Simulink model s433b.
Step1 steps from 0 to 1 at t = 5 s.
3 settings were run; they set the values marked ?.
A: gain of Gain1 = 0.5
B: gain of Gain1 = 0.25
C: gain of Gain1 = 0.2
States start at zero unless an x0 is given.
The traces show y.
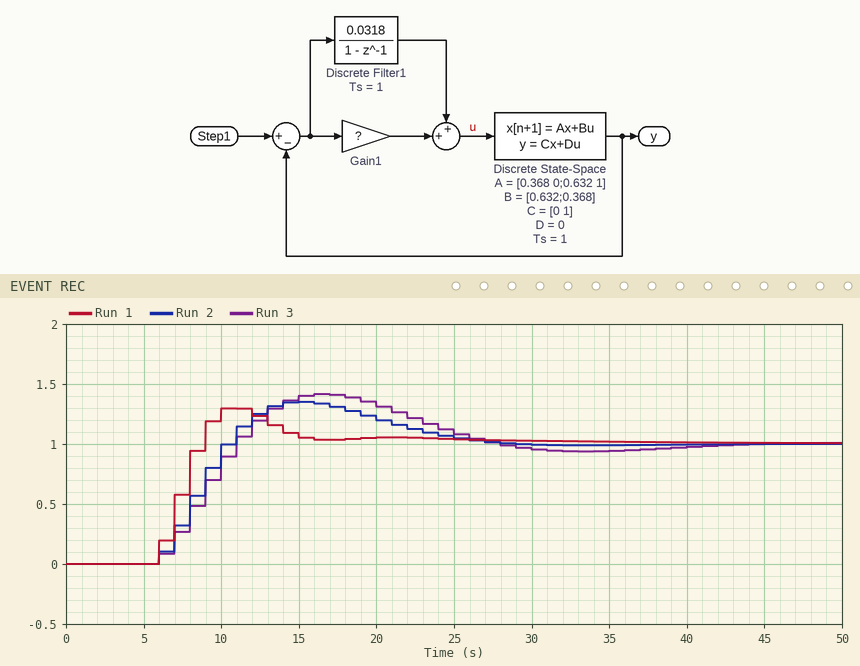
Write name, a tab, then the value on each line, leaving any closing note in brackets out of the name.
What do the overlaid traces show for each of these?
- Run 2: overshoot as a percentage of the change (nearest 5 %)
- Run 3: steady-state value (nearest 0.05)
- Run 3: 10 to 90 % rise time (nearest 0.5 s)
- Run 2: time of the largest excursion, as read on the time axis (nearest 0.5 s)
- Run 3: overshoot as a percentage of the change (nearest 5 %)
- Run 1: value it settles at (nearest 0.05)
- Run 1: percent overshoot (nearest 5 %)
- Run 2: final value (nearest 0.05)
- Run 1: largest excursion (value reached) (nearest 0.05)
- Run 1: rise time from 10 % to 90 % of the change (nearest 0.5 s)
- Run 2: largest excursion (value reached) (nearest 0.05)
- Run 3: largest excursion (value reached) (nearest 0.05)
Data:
Run 2: overshoot as a percentage of the change	35 %
Run 3: steady-state value	1.00
Run 3: 10 to 90 % rise time	4.0 s
Run 2: time of the largest excursion, as read on the time axis	15.0 s
Run 3: overshoot as a percentage of the change	40 %
Run 1: value it settles at	1.00
Run 1: percent overshoot	30 %
Run 2: final value	1.00
Run 1: largest excursion (value reached)	1.30
Run 1: rise time from 10 % to 90 % of the change	2.0 s
Run 2: largest excursion (value reached)	1.35
Run 3: largest excursion (value reached)	1.40
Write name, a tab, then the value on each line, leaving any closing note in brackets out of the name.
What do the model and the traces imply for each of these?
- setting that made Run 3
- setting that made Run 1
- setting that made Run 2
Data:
setting that made Run 3	C
setting that made Run 1	A
setting that made Run 2	B
